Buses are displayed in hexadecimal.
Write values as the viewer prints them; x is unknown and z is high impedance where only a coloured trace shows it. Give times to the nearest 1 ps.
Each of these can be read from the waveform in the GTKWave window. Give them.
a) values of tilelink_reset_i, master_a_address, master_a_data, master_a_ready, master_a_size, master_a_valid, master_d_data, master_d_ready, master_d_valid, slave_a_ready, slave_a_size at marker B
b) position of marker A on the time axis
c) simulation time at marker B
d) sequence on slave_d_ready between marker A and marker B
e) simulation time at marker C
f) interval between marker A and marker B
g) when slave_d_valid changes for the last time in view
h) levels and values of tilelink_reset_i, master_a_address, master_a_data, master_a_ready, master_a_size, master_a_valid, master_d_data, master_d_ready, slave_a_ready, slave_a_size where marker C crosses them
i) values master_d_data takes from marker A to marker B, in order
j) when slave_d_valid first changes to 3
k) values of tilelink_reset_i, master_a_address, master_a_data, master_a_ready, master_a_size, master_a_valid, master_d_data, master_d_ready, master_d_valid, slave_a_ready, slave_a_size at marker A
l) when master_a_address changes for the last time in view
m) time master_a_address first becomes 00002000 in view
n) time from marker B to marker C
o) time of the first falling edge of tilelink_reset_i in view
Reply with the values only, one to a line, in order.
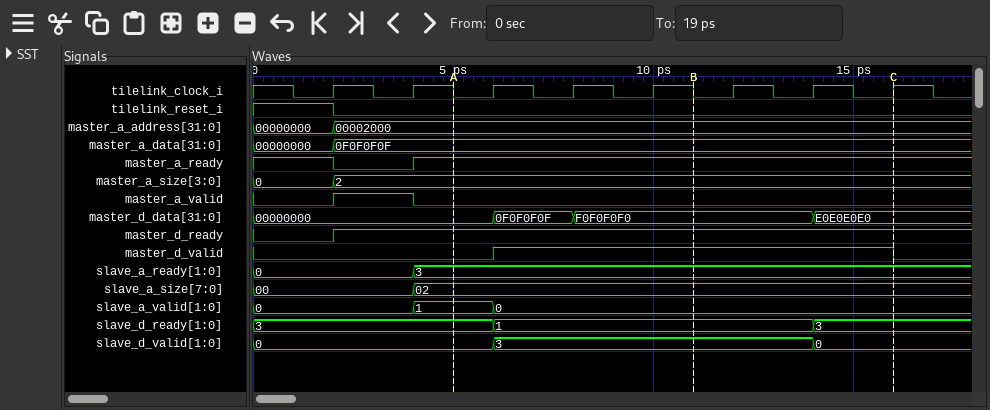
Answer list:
tilelink_reset_i=0, master_a_address=00002000, master_a_data=0F0F0F0F, master_a_ready=1, master_a_size=2, master_a_valid=0, master_d_data=F0F0F0F0, master_d_ready=1, master_d_valid=1, slave_a_ready=3, slave_a_size=02
5 ps
11 ps
3, 1
16 ps
6 ps
14 ps
tilelink_reset_i=0, master_a_address=00002000, master_a_data=0F0F0F0F, master_a_ready=1, master_a_size=2, master_a_valid=0, master_d_data=E0E0E0E0, master_d_ready=1, slave_a_ready=3, slave_a_size=02
00000000, 0F0F0F0F, F0F0F0F0
6 ps
tilelink_reset_i=0, master_a_address=00002000, master_a_data=0F0F0F0F, master_a_ready=1, master_a_size=2, master_a_valid=0, master_d_data=00000000, master_d_ready=1, master_d_valid=0, slave_a_ready=3, slave_a_size=02
2 ps
2 ps
5 ps
2 ps
